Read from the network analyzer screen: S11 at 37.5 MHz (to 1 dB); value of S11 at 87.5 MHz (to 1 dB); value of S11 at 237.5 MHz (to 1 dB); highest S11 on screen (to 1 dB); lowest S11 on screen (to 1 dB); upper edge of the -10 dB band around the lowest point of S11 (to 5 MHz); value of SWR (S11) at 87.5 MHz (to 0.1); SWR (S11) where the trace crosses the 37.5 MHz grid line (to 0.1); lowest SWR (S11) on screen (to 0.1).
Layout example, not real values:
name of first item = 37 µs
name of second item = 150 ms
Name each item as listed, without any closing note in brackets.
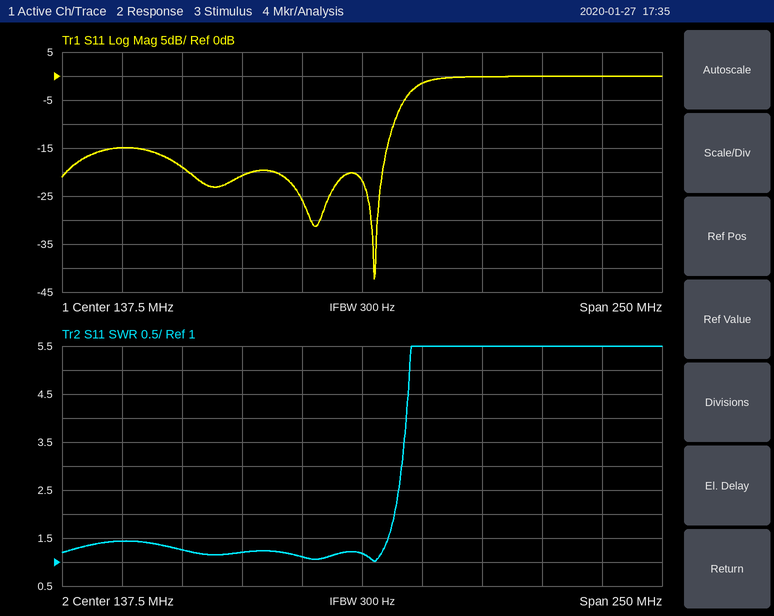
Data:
S11 at 37.5 MHz = -15 dB
value of S11 at 87.5 MHz = -21 dB
value of S11 at 237.5 MHz = 0 dB
highest S11 on screen = 0 dB
lowest S11 on screen = -42 dB
upper edge of the -10 dB band around the lowest point of S11 = 150 MHz
value of SWR (S11) at 87.5 MHz = 1.2
SWR (S11) where the trace crosses the 37.5 MHz grid line = 1.4
lowest SWR (S11) on screen = 1.0
